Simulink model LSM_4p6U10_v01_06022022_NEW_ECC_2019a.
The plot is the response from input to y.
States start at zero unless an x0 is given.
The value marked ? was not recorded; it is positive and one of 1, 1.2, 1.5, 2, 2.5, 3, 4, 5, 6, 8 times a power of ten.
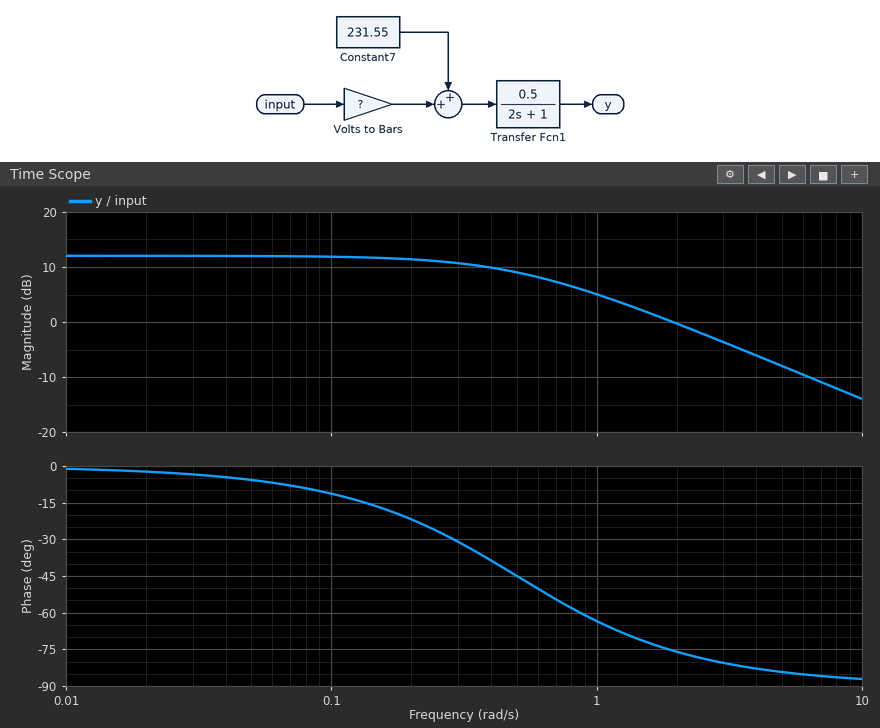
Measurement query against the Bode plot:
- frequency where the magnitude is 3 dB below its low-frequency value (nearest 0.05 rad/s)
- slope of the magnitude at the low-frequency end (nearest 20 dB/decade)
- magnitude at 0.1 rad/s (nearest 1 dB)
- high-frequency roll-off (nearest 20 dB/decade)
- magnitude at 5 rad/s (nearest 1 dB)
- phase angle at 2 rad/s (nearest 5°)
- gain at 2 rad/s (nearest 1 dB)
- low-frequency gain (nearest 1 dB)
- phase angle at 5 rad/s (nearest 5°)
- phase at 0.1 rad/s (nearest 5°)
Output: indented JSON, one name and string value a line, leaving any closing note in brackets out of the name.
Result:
{
  "frequency where the magnitude is 3 dB below its low-frequency value": "0.50 rad/s",
  "slope of the magnitude at the low-frequency end": "0 dB/decade",
  "magnitude at 0.1 rad/s": "12 dB",
  "high-frequency roll-off": "-20 dB/decade",
  "magnitude at 5 rad/s": "-8 dB",
  "phase angle at 2 rad/s": "-75°",
  "gain at 2 rad/s": "0 dB",
  "low-frequency gain": "12 dB",
  "phase angle at 5 rad/s": "-85°",
  "phase at 0.1 rad/s": "-10°"
}
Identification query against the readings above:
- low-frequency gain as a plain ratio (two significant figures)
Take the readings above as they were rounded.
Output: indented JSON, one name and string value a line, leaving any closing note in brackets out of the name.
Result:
{
  "low-frequency gain as a plain ratio": "4.0"
}
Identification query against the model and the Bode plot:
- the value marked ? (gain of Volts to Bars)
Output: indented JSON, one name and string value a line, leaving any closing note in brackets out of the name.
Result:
{
  "the value marked ?": "8"
}
